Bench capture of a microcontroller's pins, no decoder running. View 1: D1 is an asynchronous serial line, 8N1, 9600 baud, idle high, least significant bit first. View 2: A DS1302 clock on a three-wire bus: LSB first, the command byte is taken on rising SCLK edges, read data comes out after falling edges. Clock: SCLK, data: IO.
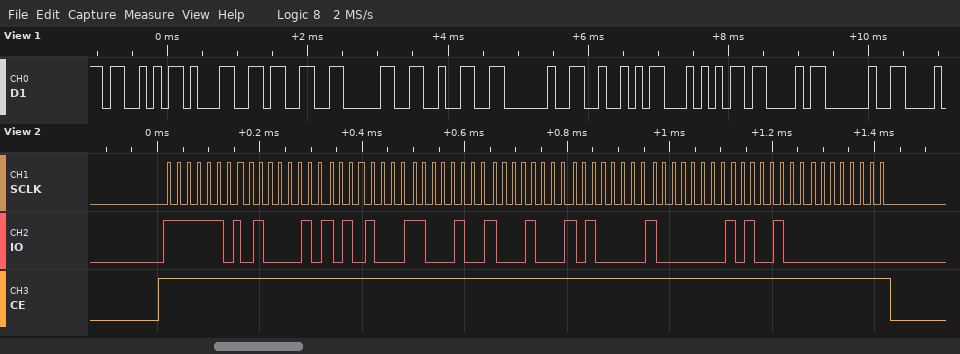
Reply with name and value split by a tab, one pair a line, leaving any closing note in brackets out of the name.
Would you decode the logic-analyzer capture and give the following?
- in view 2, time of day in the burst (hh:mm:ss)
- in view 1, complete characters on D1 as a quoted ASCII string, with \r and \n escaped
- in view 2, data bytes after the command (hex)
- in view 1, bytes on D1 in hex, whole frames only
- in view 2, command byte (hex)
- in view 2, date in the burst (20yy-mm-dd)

in view 2, time of day in the burst	23:15:42
in view 1, complete characters on D1 as a quoted ASCII string, with \r and \n escaped	"S1302 RTC "
in view 2, data bytes after the command	42 15 23 11 05 01 25 00
in view 1, bytes on D1 in hex, whole frames only	0x53 0x31 0x33 0x30 0x32 0x20 0x52 0x54 0x43 0x20
in view 2, command byte	0xBF
in view 2, date in the burst	2025-05-11
